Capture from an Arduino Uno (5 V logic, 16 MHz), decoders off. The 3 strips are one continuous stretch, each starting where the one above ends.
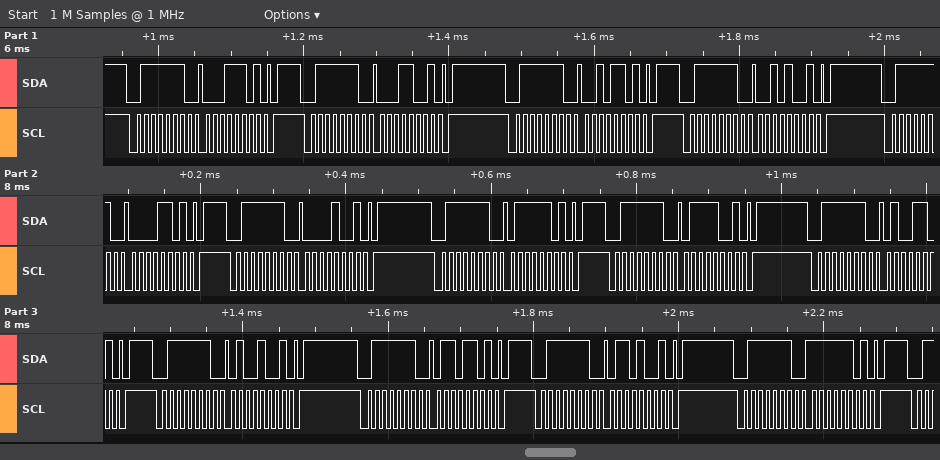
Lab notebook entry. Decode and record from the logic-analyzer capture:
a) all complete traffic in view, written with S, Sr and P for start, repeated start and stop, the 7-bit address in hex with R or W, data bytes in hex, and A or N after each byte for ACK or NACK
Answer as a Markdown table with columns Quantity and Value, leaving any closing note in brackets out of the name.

| Quantity | Value |
|---|---|
| all complete traffic in view, written with S, Sr and P for start, repeated start and stop, the 7-bit address in hex with R or W, data bytes in hex, and A or N after each byte for ACK or NACK | S 3FW A 1D A P S 3FW A 19 A P S 3FW A 2D A P S 3FW A 29 A P S 3FW A 0D A P S 3FW A 09 A P S 3FW A 7D A P S 3FW A 79 A P S 3FW A 4D A P S 3FW A 49 A P S 3FW A 6D A P S 3FW A 69 A P S 3FW A FD A P |
